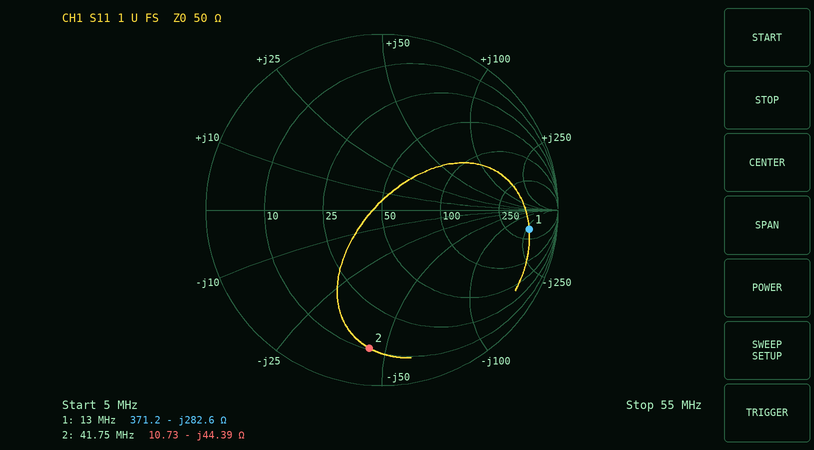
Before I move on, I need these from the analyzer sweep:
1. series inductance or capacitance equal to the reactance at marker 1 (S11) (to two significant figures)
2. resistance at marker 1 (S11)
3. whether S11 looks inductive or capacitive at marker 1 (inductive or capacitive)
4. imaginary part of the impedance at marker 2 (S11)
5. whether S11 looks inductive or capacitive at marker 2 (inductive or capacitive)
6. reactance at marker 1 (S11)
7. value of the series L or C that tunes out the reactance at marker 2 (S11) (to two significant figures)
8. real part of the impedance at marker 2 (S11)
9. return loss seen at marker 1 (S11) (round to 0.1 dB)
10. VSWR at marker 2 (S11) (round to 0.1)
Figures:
43 pF
371.2 Ω
capacitive
-44.39 Ω
capacitive
-282.6 Ω
170 nH
10.73 Ω
1.5 dB
8.4
